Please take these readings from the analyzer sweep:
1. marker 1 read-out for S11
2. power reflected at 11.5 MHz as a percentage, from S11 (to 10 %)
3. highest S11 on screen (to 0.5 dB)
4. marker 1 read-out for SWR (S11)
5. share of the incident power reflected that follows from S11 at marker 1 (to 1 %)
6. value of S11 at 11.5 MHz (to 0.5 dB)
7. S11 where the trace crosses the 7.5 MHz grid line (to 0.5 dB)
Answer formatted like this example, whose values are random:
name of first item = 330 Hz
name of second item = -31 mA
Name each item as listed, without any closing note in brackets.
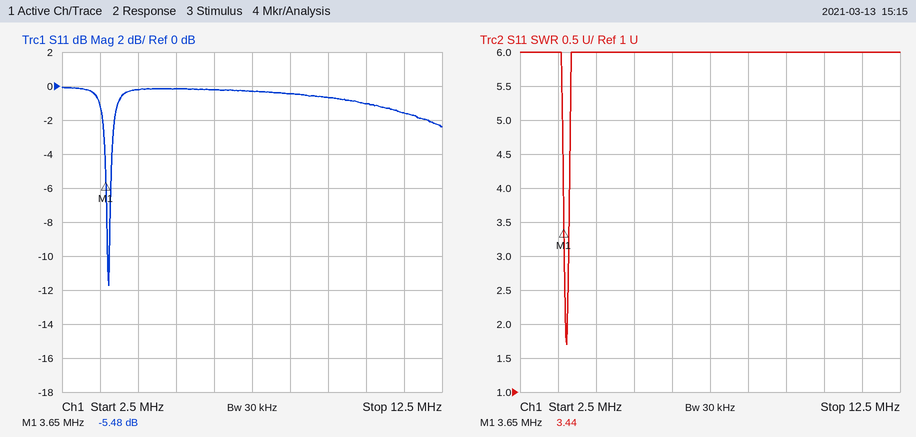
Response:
marker 1 read-out for S11 = -5.48 dB
power reflected at 11.5 MHz as a percentage, from S11 = 70 %
highest S11 on screen = 0.0 dB
marker 1 read-out for SWR = 3.44
share of the incident power reflected that follows from S11 at marker 1 = 28 %
value of S11 at 11.5 MHz = -1.5 dB
S11 where the trace crosses the 7.5 MHz grid line = -0.5 dB
